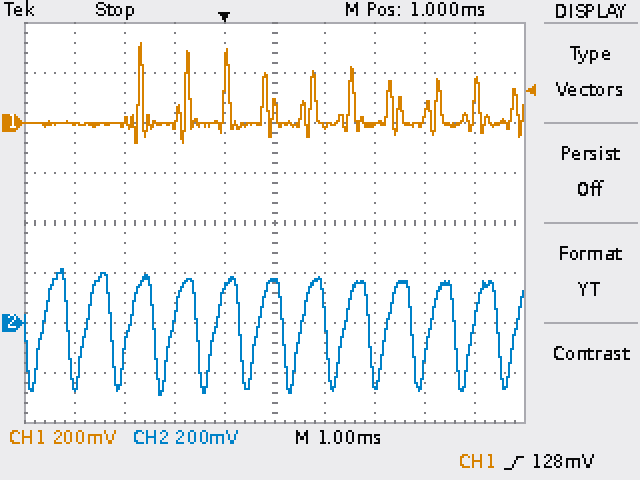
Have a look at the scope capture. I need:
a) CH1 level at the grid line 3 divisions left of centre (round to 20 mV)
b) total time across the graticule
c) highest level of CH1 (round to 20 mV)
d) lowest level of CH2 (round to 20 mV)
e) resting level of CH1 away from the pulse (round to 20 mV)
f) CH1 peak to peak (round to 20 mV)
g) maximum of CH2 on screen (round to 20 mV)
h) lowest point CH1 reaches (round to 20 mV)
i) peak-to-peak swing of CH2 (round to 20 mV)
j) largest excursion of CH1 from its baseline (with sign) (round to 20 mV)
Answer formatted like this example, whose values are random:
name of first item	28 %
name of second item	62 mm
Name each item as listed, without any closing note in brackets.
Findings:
CH1 level at the grid line 3 divisions left of centre	0 mV
total time across the graticule	10 ms
highest level of CH1	320 mV
lowest level of CH2	-280 mV
resting level of CH1 away from the pulse	0 mV
CH1 peak to peak	400 mV
maximum of CH2 on screen	220 mV
lowest point CH1 reaches	-80 mV
peak-to-peak swing of CH2	500 mV
largest excursion of CH1 from its baseline (with sign)	+320 mV
